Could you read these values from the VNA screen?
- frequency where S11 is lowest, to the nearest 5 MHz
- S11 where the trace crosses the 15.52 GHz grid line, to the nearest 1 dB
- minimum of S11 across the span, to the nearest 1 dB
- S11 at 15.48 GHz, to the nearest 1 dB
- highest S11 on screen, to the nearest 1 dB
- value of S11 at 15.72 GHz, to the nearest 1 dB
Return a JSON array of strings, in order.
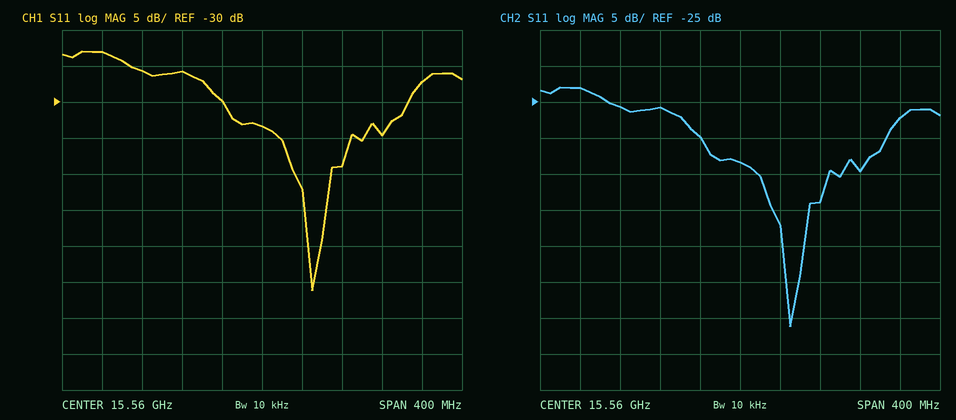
["15.610 GHz", "-30 dB", "-56 dB", "-26 dB", "-23 dB", "-27 dB"]
